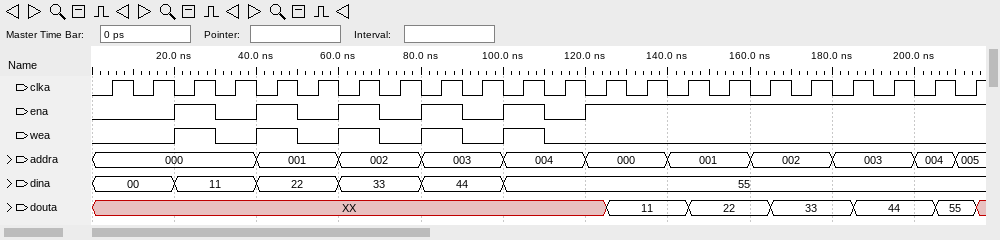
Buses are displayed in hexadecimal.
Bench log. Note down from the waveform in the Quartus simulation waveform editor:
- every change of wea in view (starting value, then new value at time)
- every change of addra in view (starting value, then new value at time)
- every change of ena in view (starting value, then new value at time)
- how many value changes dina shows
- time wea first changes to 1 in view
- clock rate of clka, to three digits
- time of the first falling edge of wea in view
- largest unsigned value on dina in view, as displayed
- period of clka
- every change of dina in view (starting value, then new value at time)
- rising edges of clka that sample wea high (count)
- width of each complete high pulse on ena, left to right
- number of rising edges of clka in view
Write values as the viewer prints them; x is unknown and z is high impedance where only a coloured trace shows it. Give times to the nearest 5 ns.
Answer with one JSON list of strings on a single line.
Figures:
["0, 1 at 20 ns, 0 at 30 ns, 1 at 40 ns, 0 at 50 ns, 1 at 60 ns, 0 at 70 ns, 1 at 80 ns, 0 at 90 ns, 1 at 100 ns, 0 at 110 ns", "000, 001 at 40 ns, 002 at 60 ns, 003 at 80 ns, 004 at 100 ns, 000 at 120 ns, 001 at 140 ns, 002 at 160 ns, 003 at 180 ns, 004 at 200 ns, 005 at 210 ns", "0, 1 at 20 ns, 0 at 30 ns, 1 at 40 ns, 0 at 50 ns, 1 at 60 ns, 0 at 70 ns, 1 at 80 ns, 0 at 90 ns, 1 at 100 ns, 0 at 110 ns, 1 at 120 ns", "5", "20 ns", "100 MHz", "30 ns", "55", "10 ns", "00, 11 at 20 ns, 22 at 40 ns, 33 at 60 ns, 44 at 80 ns, 55 at 100 ns", "5", "10 ns, 10 ns, 10 ns, 10 ns, 10 ns", "22"]
